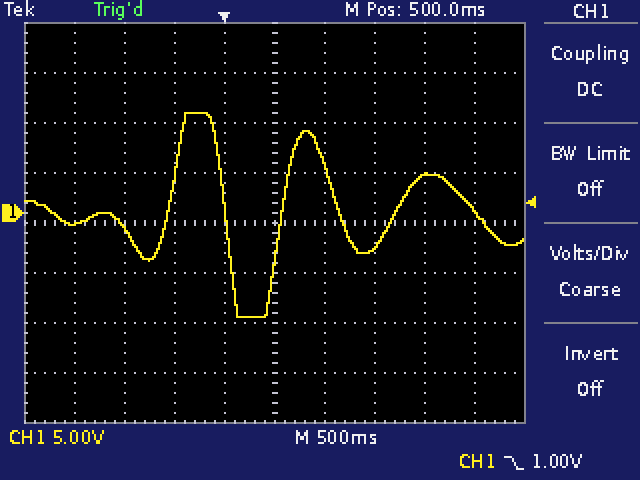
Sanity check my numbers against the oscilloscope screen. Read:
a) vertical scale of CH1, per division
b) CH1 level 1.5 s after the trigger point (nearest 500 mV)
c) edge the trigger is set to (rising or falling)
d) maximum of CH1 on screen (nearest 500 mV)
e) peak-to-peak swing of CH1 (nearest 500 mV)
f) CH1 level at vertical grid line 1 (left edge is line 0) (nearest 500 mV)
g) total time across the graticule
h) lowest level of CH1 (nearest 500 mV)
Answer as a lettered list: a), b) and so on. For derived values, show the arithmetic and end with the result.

a) 5 V
b) -3.5 V
c) falling
d) 10.0 V
e) 10.0 V − (-10.5 V) = 20.5 V
f) -1.0 V
g) 5 s
h) -10.5 V
